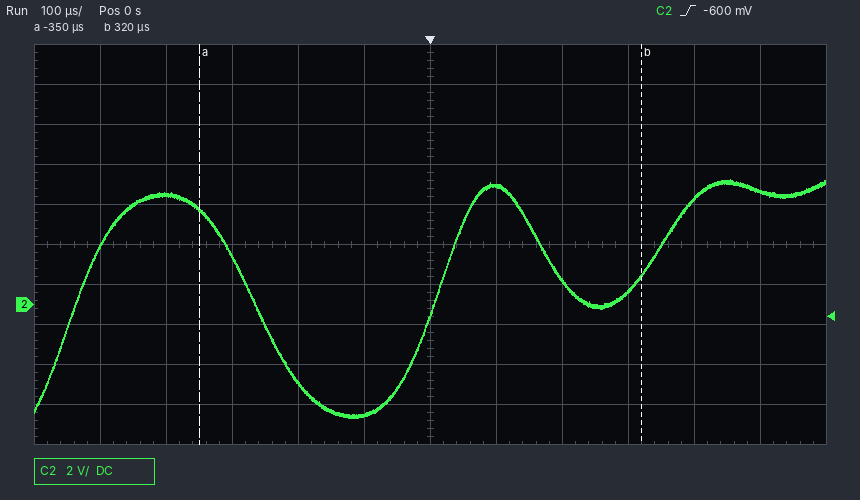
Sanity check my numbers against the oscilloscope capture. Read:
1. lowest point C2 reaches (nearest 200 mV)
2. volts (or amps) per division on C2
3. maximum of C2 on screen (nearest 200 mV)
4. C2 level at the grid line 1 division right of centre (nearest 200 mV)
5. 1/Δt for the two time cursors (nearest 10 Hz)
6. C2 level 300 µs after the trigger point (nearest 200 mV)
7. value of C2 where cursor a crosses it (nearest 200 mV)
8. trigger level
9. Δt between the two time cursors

-5.6 V
2 V
6.2 V
6.0 V
1.49 kHz
600 mV
4.8 V
-600 mV
670 µs
